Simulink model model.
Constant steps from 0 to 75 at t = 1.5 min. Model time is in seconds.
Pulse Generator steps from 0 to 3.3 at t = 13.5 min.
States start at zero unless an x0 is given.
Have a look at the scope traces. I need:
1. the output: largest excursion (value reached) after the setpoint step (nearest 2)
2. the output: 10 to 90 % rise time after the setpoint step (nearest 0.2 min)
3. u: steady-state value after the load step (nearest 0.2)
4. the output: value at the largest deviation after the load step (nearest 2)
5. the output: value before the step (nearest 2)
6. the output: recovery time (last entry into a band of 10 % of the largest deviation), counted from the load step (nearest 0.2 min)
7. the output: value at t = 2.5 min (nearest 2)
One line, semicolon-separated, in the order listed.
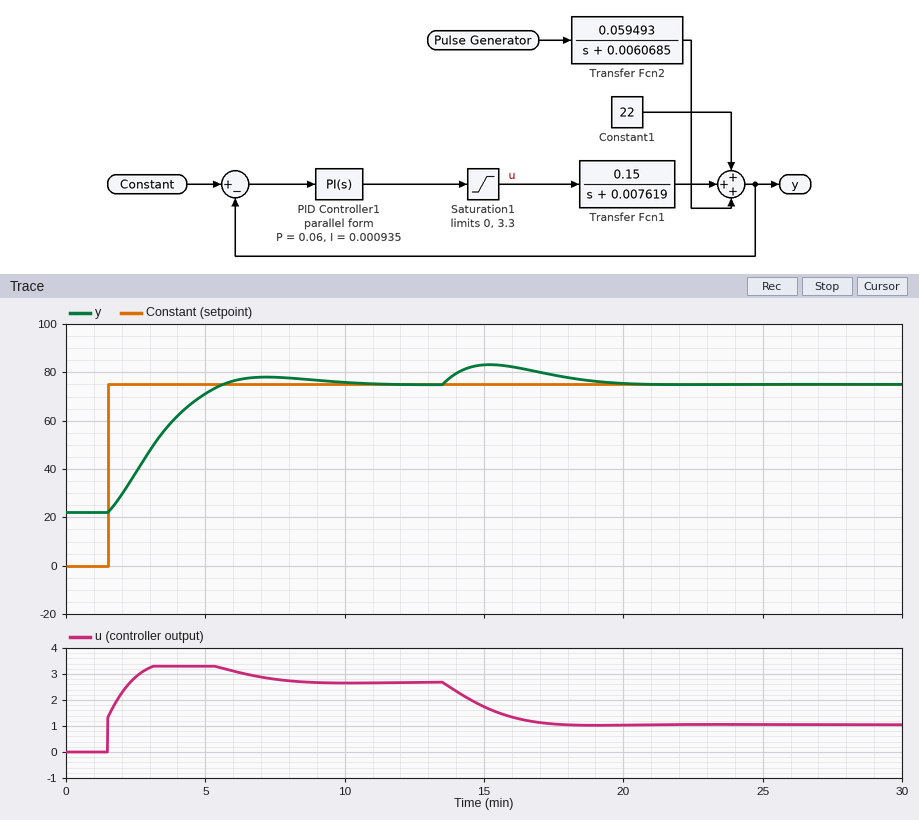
78; 3.0 min; 1.0; 84; 22; 6.0 min; 38
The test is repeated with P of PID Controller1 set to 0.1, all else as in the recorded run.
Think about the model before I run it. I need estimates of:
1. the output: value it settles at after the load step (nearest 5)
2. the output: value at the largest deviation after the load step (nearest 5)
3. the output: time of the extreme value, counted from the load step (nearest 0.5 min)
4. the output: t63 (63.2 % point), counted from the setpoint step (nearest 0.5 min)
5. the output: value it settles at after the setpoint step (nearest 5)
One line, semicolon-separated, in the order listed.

75; 80; 1.5 min; 1.5 min; 75
